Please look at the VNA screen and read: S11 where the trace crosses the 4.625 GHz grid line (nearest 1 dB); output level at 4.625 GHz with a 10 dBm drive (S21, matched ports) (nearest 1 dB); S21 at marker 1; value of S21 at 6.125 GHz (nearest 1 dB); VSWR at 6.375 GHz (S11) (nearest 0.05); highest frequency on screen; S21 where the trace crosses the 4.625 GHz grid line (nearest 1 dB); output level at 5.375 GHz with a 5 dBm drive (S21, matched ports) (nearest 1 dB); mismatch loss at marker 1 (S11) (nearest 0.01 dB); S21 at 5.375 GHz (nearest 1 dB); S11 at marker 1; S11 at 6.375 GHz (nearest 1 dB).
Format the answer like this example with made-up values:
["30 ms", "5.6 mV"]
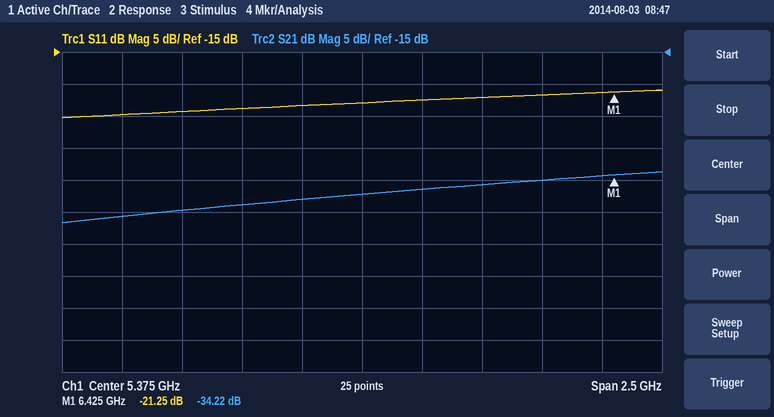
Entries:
["-24 dB", "-30 dBm", "-34.22 dB", "-35 dB", "1.20", "6.625 GHz", "-40 dB", "-32 dBm", "0.03 dB", "-37 dB", "-21.25 dB", "-21 dB"]
